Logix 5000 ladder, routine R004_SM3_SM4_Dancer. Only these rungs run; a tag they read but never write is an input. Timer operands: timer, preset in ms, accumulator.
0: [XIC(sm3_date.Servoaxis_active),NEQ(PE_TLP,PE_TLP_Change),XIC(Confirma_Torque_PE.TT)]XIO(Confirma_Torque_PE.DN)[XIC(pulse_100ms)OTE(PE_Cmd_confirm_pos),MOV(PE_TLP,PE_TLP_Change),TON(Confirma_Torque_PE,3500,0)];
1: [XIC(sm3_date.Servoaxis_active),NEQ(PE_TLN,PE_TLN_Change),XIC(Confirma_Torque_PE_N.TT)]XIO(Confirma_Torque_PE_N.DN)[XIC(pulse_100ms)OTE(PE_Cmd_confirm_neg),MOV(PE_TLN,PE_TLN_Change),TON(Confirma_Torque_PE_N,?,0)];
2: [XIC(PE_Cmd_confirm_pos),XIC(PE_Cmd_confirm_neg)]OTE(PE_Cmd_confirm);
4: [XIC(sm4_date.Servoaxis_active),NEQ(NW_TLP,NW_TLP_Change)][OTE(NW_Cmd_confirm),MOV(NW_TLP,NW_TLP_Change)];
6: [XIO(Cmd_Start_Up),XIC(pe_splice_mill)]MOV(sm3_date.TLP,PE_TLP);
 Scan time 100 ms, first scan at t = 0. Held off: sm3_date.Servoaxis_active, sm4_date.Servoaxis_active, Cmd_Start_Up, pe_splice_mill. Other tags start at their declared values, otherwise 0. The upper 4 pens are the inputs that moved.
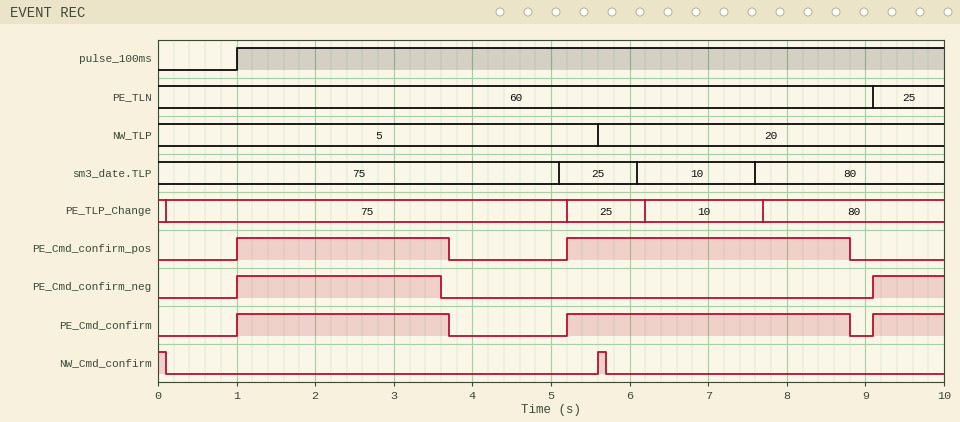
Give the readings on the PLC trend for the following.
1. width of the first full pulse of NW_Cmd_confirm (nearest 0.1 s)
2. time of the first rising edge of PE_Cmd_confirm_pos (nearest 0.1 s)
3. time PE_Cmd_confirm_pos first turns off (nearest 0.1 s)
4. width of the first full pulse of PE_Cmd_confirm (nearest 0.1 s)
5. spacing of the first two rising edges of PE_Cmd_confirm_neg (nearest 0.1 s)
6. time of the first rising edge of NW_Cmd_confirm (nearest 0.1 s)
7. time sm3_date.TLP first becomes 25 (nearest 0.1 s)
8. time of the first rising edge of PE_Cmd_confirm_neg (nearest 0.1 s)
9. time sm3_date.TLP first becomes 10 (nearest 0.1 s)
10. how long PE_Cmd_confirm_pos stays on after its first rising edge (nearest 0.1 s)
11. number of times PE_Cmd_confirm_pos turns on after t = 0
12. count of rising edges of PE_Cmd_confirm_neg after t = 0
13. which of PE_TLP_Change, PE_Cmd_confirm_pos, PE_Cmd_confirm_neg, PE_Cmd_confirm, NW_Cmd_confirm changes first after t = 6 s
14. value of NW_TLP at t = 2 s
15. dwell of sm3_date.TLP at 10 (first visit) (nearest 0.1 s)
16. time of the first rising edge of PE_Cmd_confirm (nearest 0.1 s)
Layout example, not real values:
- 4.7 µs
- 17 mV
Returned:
- 0.1 s
- 1.0 s
- 3.7 s
- 2.7 s
- 8.1 s
- 5.6 s
- 5.1 s
- 1.0 s
- 6.1 s
- 2.7 s
- 2
- 2
- PE_TLP_Change
- 5
- 1.5 s
- 1.0 s
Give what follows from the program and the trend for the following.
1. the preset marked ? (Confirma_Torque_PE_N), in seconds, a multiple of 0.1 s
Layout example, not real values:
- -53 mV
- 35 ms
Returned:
- 3.5 s
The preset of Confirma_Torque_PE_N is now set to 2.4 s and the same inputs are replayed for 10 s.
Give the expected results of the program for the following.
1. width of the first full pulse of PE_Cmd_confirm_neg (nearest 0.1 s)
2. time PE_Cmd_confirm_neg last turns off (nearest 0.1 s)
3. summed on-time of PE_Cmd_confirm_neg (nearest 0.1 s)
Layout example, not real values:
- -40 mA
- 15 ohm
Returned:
- 1.5 s
- 2.5 s
- 2.4 s
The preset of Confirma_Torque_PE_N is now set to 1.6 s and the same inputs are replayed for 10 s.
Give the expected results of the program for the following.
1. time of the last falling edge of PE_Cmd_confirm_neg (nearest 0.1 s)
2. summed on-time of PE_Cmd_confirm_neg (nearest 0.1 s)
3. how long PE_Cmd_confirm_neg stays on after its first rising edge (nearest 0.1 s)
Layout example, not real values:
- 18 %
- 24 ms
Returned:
- 1.7 s
- 1.6 s
- 0.7 s
